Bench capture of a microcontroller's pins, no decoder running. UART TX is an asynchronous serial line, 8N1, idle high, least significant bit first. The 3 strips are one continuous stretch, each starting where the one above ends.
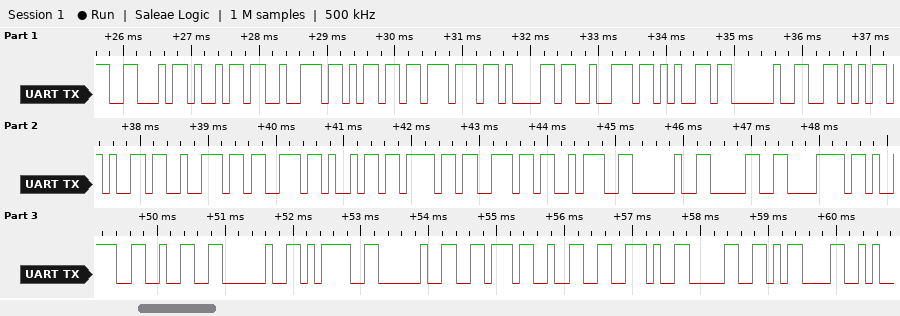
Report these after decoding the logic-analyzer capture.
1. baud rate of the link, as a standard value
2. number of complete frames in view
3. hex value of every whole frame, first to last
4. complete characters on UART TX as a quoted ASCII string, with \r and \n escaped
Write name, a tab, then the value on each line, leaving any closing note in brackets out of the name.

baud rate of the link, as a standard value	9600 baud
number of complete frames in view	30
hex value of every whole frame, first to last	46 69 72 6D 77 61 72 65 20 56 65 72 73 69 6F 6E 3A 20 30 78 39 32 20 3D 20 76 32 2E 30 0D
complete characters on UART TX as a quoted ASCII string, with \r and \n escaped	"Firmware Version: 0x92 = v2.0\r"
